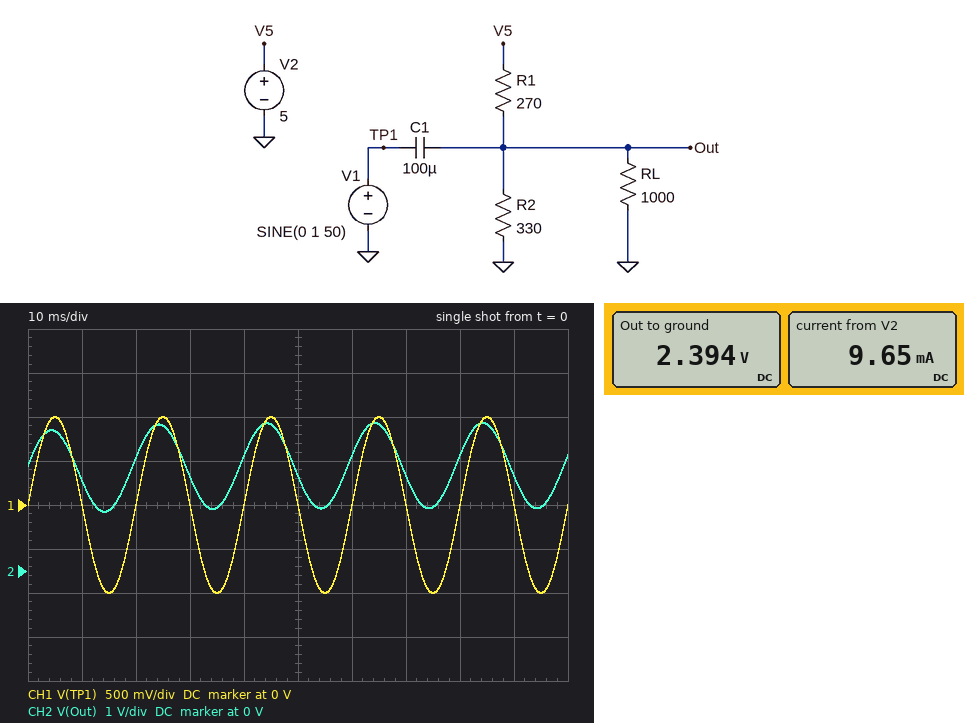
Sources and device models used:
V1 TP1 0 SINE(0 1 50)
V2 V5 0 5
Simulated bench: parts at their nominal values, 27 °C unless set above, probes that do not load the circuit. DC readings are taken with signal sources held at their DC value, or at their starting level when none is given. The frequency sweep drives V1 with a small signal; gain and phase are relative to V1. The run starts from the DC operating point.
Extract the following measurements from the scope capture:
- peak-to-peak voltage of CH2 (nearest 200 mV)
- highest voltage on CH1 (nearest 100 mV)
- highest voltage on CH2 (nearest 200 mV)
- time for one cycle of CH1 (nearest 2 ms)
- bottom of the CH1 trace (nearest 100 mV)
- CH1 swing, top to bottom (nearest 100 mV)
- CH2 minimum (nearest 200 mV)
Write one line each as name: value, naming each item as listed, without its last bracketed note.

peak-to-peak voltage of CH2: 2.0 V
highest voltage on CH1: 1.0 V
highest voltage on CH2: 3.4 V
time for one cycle of CH1: 20 ms
bottom of the CH1 trace: -1.0 V
CH1 swing, top to bottom: 2.0 V
CH2 minimum: 1.4 V
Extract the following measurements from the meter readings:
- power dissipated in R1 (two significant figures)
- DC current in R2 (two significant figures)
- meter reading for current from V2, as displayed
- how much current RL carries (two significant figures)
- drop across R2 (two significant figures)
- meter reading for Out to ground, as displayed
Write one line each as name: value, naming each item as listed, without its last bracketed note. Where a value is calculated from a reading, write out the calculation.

power dissipated in R1: (5 V - 2.394 V)^2 / 270 Ω = 25 mW
DC current in R2: (2.394 V) / 330 Ω = 7.3 mA
meter reading for current from V2, as displayed: 9.65 mA
how much current RL carries: (2.394 V) / 1 kΩ = 2.4 mA
drop across R2: 2.394 V = 2.4 V
meter reading for Out to ground, as displayed: 2.394 V
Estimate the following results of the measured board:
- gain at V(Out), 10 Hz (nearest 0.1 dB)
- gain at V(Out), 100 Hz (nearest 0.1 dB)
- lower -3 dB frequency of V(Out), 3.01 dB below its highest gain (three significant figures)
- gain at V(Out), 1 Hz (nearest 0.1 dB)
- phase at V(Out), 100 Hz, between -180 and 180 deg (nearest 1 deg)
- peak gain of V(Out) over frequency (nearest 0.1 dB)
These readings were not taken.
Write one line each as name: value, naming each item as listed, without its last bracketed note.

gain at V(Out), 10 Hz: -4.0 dB
gain at V(Out), 100 Hz: -0.1 dB
lower -3 dB frequency of V(Out), 3.01 dB below its highest gain: 12.3 Hz
gain at V(Out), 1 Hz: -21.8 dB
phase at V(Out), 100 Hz, between -180 and 180 deg: 7 deg
peak gain of V(Out) over frequency: 0 dB
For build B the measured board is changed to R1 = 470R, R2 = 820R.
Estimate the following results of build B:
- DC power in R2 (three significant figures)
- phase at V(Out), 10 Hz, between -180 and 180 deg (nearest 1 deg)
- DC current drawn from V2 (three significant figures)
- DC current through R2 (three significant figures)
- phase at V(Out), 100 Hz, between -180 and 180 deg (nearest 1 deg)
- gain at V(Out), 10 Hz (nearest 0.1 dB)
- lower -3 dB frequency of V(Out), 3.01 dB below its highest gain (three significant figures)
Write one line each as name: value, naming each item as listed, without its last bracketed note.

DC power in R2: 7.30 mW
phase at V(Out), 10 Hz, between -180 and 180 deg: 35 deg
DC current drawn from V2: 5.43 mA
DC current through R2: 2.98 mA
phase at V(Out), 100 Hz, between -180 and 180 deg: 4 deg
gain at V(Out), 10 Hz: -1.7 dB
lower -3 dB frequency of V(Out), 3.01 dB below its highest gain: 6.92 Hz
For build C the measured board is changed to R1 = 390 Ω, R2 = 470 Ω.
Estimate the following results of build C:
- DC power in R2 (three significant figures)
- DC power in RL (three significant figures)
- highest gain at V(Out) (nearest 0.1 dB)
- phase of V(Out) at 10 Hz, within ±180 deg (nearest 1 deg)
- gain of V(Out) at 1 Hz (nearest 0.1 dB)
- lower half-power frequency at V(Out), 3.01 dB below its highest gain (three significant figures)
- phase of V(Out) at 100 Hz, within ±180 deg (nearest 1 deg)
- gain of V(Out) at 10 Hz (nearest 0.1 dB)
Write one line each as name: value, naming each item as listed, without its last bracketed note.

DC power in R2: 10.8 mW
DC power in RL: 5.07 mW
highest gain at V(Out): 0 dB
phase of V(Out) at 10 Hz, within ±180 deg: 42 deg
gain of V(Out) at 1 Hz: -19.2 dB
lower half-power frequency at V(Out), 3.01 dB below its highest gain: 9.06 Hz
phase of V(Out) at 100 Hz, within ±180 deg: 5 deg
gain of V(Out) at 10 Hz: -2.6 dB
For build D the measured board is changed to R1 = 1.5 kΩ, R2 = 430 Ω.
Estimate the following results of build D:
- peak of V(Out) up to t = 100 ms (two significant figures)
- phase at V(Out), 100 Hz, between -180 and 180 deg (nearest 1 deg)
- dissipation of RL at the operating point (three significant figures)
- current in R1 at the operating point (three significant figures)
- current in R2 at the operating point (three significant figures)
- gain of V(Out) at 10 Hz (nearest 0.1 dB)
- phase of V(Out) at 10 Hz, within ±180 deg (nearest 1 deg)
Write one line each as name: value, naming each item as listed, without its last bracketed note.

peak of V(Out) up to t = 100 ms: 1.8 V
phase at V(Out), 100 Hz, between -180 and 180 deg: 4 deg
dissipation of RL at the operating point: 697 µW
current in R1 at the operating point: 2.78 mA
current in R2 at the operating point: 1.94 mA
gain of V(Out) at 10 Hz: -1.5 dB
phase of V(Out) at 10 Hz, within ±180 deg: 32 deg
